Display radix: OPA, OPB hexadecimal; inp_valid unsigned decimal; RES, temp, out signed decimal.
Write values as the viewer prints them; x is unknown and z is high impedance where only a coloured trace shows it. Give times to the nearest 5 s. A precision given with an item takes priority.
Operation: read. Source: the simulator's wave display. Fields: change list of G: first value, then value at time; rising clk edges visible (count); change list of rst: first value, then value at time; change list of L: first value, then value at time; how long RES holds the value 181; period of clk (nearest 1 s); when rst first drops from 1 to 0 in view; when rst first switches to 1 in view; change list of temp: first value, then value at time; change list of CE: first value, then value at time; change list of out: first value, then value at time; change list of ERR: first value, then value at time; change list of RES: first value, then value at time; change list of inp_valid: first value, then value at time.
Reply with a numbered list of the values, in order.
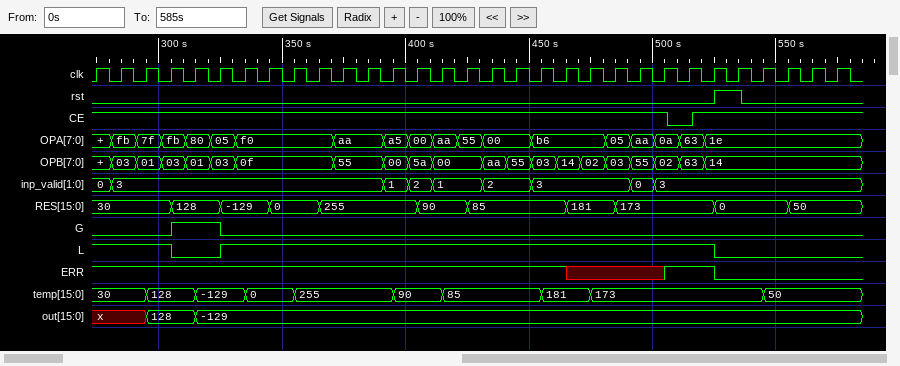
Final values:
1. 0, 1 at 305 s, 0 at 325 s
2. 31
3. 0, 1 at 525 s, 0 at 535 s
4. 1, 0 at 305 s, 1 at 325 s, 0 at 525 s
5. 20 s
6. 10 s
7. 535 s
8. 525 s
9. 30, 128 at 295 s, -129 at 315 s, 0 at 335 s, 255 at 355 s, 90 at 395 s, 85 at 415 s, 181 at 455 s, 173 at 475 s, 50 at 545 s
10. 1, 0 at 505 s, 1 at 515 s
11. x, 128 at 295 s, -129 at 315 s
12. 1, x at 465 s, 1 at 505 s, 0 at 525 s
13. 30, 128 at 305 s, -129 at 325 s, 0 at 345 s, 255 at 365 s, 90 at 405 s, 85 at 425 s, 181 at 465 s, 173 at 485 s, 0 at 525 s, 50 at 555 s
14. 0, 3 at 280 s, 1 at 390 s, 2 at 400 s, 1 at 410 s, 2 at 430 s, 3 at 450 s, 0 at 490 s, 3 at 500 s
